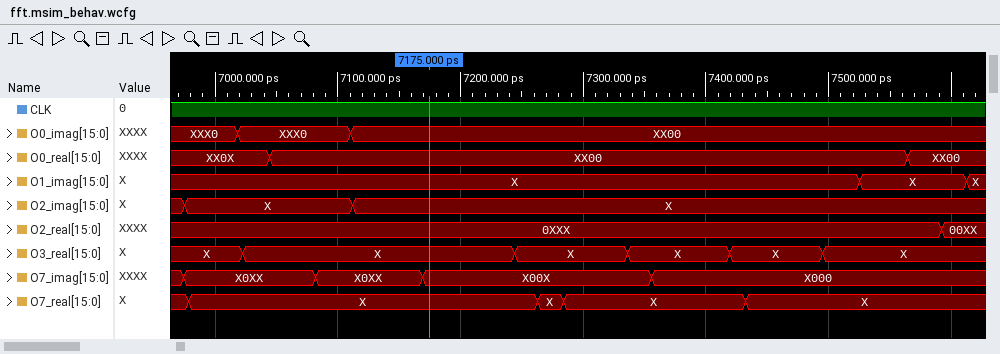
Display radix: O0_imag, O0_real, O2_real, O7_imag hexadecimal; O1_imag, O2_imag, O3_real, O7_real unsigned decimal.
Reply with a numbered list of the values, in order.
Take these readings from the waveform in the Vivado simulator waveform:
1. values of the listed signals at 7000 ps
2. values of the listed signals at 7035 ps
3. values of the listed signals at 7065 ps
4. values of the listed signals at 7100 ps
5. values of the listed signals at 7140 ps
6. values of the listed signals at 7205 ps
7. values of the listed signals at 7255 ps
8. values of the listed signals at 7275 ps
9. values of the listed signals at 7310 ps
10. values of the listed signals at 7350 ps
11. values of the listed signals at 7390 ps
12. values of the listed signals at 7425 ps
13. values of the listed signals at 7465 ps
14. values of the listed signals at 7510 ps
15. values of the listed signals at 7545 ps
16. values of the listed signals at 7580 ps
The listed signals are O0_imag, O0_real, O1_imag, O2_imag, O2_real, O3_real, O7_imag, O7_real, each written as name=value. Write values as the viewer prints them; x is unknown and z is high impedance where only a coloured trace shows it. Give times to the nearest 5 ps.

1. O0_imag=XXX0, O0_real=XX0X, O1_imag=X, O2_imag=X, O2_real=0XXX, O3_real=X, O7_imag=X0XX, O7_real=X
2. O0_imag=XXX0, O0_real=XX0X, O1_imag=X, O2_imag=X, O2_real=0XXX, O3_real=X, O7_imag=X0XX, O7_real=X
3. O0_imag=XXX0, O0_real=XX00, O1_imag=X, O2_imag=X, O2_real=0XXX, O3_real=X, O7_imag=X0XX, O7_real=X
4. O0_imag=XXX0, O0_real=XX00, O1_imag=X, O2_imag=X, O2_real=0XXX, O3_real=X, O7_imag=X0XX, O7_real=X
5. O0_imag=XX00, O0_real=XX00, O1_imag=X, O2_imag=X, O2_real=0XXX, O3_real=X, O7_imag=X0XX, O7_real=X
6. O0_imag=XX00, O0_real=XX00, O1_imag=X, O2_imag=X, O2_real=0XXX, O3_real=X, O7_imag=X00X, O7_real=X
7. O0_imag=XX00, O0_real=XX00, O1_imag=X, O2_imag=X, O2_real=0XXX, O3_real=X, O7_imag=X00X, O7_real=X
8. O0_imag=XX00, O0_real=XX00, O1_imag=X, O2_imag=X, O2_real=0XXX, O3_real=X, O7_imag=X00X, O7_real=X
9. O0_imag=XX00, O0_real=XX00, O1_imag=X, O2_imag=X, O2_real=0XXX, O3_real=X, O7_imag=X00X, O7_real=X
10. O0_imag=XX00, O0_real=XX00, O1_imag=X, O2_imag=X, O2_real=0XXX, O3_real=X, O7_imag=X00X, O7_real=X
11. O0_imag=XX00, O0_real=XX00, O1_imag=X, O2_imag=X, O2_real=0XXX, O3_real=X, O7_imag=X000, O7_real=X
12. O0_imag=XX00, O0_real=XX00, O1_imag=X, O2_imag=X, O2_real=0XXX, O3_real=X, O7_imag=X000, O7_real=X
13. O0_imag=XX00, O0_real=XX00, O1_imag=X, O2_imag=X, O2_real=0XXX, O3_real=X, O7_imag=X000, O7_real=X
14. O0_imag=XX00, O0_real=XX00, O1_imag=X, O2_imag=X, O2_real=0XXX, O3_real=X, O7_imag=X000, O7_real=X
15. O0_imag=XX00, O0_real=XX00, O1_imag=X, O2_imag=X, O2_real=0XXX, O3_real=X, O7_imag=X000, O7_real=X
16. O0_imag=XX00, O0_real=XX00, O1_imag=X, O2_imag=X, O2_real=0XXX, O3_real=X, O7_imag=X000, O7_real=X
